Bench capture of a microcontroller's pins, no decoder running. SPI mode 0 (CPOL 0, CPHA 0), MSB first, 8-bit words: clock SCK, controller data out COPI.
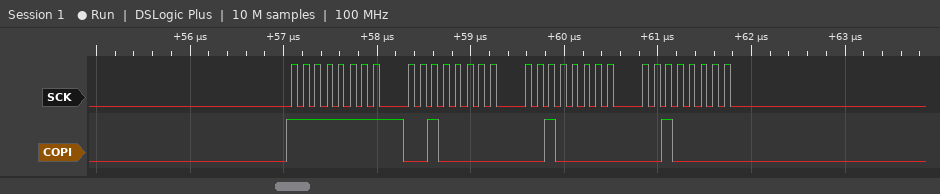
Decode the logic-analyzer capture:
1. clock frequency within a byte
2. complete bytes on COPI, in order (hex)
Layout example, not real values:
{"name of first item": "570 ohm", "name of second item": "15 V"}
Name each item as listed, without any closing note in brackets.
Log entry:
{"clock frequency within a byte": "8 MHz", "complete bytes on COPI, in order": "FF 20 20 20"}
